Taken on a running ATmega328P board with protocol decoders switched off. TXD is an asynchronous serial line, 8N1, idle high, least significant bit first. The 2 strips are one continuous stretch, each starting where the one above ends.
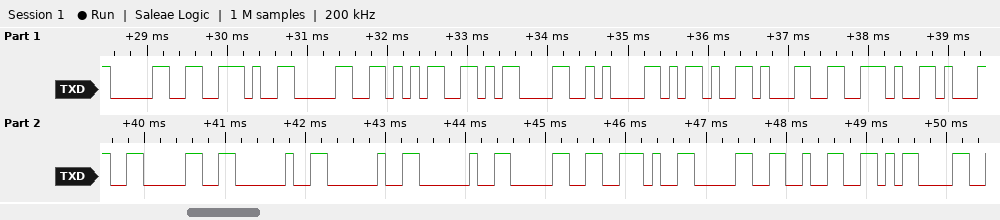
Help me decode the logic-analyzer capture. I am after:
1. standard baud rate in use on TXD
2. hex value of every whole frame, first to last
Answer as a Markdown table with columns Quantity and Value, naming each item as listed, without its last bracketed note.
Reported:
| Quantity | Value |
|---|---|
| standard baud rate in use on TXD | 9600 baud |
| hex value of every whole frame, first to last | 0x30 0x2E 0x30 0x35 0x0D 0x0A 0x2D 0x31 0x2E 0x31 0x30 0x20 0x20 0x20 0x30 0x2E 0x30 0x32 0x0D |
